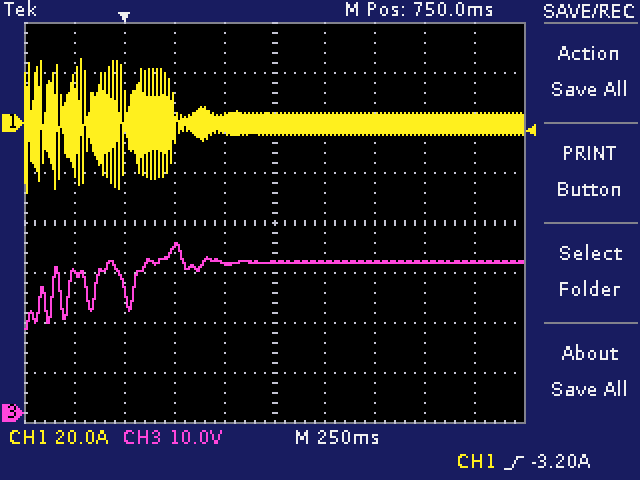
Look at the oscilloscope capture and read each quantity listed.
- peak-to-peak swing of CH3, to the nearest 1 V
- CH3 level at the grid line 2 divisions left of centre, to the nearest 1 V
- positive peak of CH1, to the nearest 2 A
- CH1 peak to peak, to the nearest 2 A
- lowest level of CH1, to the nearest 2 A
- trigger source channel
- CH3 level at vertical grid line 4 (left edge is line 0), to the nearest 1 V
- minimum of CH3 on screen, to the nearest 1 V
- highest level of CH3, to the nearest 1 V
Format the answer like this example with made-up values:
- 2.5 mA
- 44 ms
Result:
- 17 V
- 33 V
- 26 A
- 54 A
- -28 A
- CH1
- 30 V
- 17 V
- 34 V
